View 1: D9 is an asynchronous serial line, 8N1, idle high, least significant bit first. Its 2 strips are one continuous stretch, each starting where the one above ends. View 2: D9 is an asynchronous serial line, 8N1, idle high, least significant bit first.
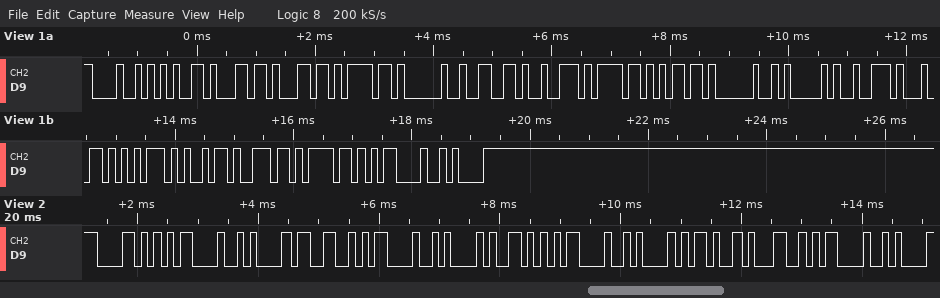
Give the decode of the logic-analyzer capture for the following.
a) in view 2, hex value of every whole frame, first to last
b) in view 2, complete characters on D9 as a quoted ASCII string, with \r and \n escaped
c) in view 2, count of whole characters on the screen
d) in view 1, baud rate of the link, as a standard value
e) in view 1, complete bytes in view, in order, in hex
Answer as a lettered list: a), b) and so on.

a) 0x58 0x0D 0x0A 0x33 0x0D 0x0A 0x59 0x0D 0x0A 0x2D 0x31 0x0D 0x0A
b) "X\r\n3\r\nY\r\n-1\r\n"
c) 13
d) 9600 baud
e) 48 65 6C 6C 6F 20 66 72 6F 6D 20 41 72 64 75 69 6E 6F 0D 0A
